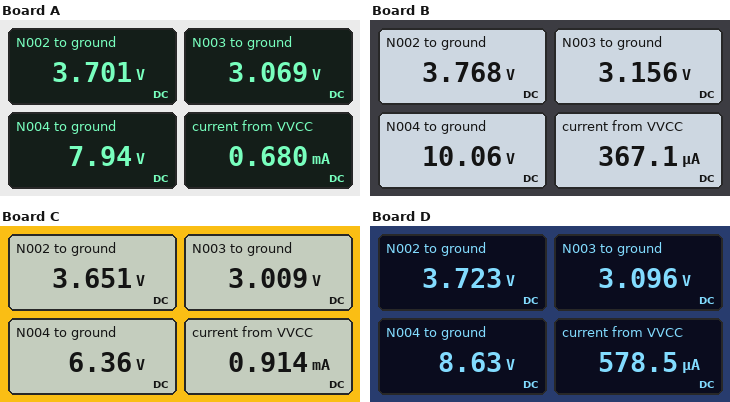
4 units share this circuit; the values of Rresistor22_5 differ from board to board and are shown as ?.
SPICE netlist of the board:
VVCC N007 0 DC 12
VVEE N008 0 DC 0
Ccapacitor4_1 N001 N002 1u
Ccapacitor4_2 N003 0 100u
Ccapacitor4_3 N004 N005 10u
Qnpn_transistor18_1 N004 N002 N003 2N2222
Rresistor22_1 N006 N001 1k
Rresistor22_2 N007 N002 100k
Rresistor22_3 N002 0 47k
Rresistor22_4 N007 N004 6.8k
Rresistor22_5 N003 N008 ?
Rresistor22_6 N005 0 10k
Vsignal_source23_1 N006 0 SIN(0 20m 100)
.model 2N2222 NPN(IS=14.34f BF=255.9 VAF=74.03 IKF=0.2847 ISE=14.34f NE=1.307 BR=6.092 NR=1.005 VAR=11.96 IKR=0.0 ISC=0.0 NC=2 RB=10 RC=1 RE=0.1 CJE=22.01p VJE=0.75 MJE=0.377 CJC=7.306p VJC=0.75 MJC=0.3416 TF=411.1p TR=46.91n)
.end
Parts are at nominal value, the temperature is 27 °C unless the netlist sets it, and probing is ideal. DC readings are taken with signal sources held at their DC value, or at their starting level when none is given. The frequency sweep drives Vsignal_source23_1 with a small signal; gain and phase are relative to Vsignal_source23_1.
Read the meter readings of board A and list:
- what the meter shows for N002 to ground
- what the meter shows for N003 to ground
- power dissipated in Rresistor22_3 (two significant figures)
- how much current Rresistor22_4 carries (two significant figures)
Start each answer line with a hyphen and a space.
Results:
- 3.701 V
- 3.069 V
- 290 µW
- 600 µA
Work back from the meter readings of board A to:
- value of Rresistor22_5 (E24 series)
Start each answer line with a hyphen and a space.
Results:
- 5.1 kΩ
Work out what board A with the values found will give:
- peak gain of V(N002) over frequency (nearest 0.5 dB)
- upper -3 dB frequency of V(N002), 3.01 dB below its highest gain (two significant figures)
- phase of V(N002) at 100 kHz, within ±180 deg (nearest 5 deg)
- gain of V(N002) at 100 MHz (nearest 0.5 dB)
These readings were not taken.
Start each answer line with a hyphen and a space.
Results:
- -1.5 dB
- 460 kHz
- -10 deg
- -30.0 dB
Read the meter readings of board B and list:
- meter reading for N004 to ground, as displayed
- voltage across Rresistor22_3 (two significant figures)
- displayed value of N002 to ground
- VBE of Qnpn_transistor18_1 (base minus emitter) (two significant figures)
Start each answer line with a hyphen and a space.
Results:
- 10.06 V
- 3.8 V
- 3.768 V
- 610 mV
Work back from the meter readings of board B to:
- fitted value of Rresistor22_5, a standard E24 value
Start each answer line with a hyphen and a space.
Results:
- 11 kΩ
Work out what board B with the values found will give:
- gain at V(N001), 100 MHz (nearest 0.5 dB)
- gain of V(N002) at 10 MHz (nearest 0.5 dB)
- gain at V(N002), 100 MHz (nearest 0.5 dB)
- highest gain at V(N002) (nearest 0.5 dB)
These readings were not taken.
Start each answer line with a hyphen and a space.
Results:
- -28.0 dB
- -19.5 dB
- -28.0 dB
- -1.0 dB
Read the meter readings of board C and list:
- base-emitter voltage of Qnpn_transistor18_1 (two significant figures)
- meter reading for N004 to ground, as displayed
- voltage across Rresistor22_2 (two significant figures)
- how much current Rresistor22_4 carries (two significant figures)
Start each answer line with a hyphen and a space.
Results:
- 640 mV
- 6.36 V
- 8.3 V
- 830 µA
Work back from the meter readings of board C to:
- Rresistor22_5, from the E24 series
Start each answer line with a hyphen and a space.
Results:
- 3.6 kΩ
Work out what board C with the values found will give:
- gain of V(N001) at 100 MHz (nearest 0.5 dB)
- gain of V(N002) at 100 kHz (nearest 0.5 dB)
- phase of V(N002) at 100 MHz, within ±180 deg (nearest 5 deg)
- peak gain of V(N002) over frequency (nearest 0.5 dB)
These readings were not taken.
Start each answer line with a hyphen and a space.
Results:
- -31.0 dB
- -2.0 dB
- -30 deg
- -2.0 dB
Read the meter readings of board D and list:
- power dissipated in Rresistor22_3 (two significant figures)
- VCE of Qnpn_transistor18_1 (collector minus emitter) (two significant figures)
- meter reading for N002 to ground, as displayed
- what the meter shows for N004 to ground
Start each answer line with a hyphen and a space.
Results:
- 290 µW
- 5.5 V
- 3.723 V
- 8.63 V
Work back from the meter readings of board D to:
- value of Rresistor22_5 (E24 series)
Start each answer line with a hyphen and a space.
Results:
- 6.2 kΩ
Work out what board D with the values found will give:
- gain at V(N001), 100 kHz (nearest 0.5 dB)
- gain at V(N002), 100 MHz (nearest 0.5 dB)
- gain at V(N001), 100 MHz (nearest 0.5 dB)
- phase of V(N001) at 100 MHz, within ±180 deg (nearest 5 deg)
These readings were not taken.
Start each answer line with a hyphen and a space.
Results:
- -1.5 dB
- -29.5 dB
- -29.5 dB
- -40 deg
